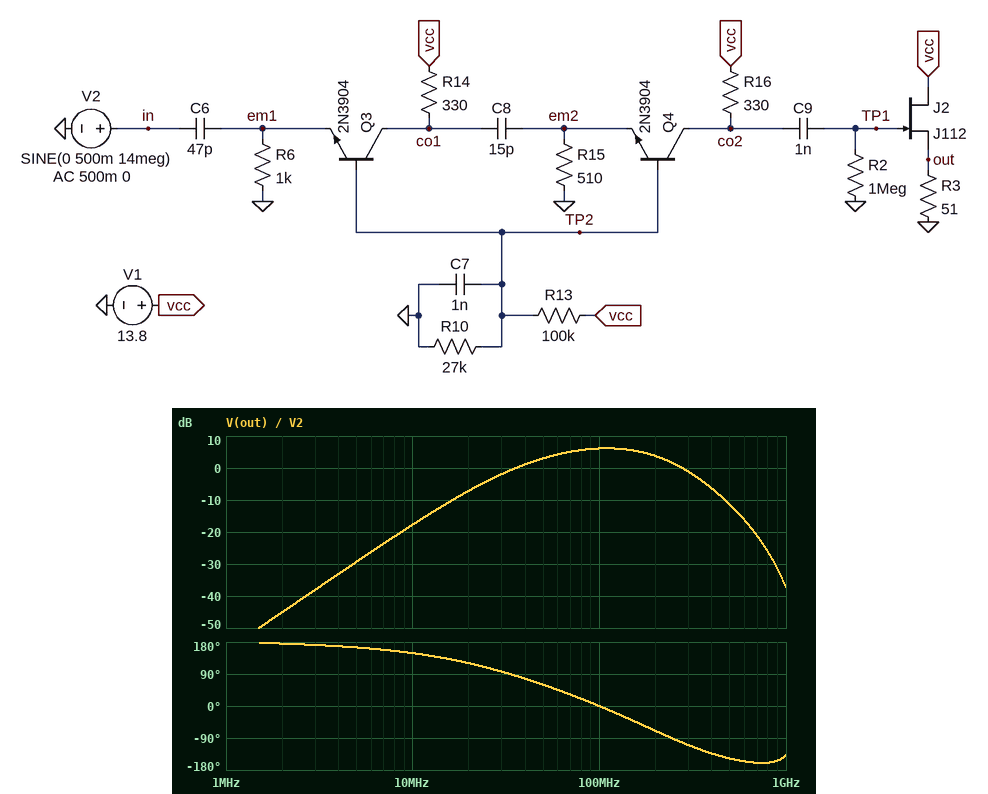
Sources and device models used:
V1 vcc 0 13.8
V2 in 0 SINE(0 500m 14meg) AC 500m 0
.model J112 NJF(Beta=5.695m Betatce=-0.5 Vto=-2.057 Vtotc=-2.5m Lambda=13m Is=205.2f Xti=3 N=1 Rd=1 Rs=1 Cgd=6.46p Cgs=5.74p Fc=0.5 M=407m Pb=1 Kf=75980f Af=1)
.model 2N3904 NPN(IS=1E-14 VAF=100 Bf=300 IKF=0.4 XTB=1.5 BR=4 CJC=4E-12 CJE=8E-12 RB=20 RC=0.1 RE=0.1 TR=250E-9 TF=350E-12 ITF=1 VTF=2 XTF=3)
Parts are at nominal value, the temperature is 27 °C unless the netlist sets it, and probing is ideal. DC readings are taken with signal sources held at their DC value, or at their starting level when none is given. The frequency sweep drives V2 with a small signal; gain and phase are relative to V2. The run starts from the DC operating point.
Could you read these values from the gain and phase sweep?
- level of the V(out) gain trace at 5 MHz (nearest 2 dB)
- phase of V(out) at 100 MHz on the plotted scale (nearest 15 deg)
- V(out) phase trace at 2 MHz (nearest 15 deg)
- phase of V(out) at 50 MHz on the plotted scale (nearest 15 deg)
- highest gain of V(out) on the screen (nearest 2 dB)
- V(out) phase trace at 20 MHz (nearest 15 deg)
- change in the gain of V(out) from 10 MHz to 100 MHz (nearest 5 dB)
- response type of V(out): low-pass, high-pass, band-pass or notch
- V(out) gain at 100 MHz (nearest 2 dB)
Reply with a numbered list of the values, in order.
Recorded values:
1. -30 dB
2. 0 deg
3. 180 deg
4. 60 deg
5. 6 dB
6. 120 deg
7. 25 dB
8. band-pass
9. 6 dB
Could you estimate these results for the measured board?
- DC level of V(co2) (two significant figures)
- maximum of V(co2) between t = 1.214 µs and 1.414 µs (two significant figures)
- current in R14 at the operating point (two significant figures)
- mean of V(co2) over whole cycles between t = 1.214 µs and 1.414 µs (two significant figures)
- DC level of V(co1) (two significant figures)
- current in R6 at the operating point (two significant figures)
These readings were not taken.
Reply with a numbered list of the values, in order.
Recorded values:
1. 13 V
2. 13 V
3. 1.9 mA
4. 13 V
5. 13 V
6. 1.9 mA
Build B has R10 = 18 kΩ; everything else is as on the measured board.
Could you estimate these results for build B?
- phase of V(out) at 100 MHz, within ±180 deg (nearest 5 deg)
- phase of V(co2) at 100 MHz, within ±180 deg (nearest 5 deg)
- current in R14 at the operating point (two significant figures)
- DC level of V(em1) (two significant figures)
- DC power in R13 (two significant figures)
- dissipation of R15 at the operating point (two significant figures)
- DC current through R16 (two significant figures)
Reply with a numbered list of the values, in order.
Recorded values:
1. -10 deg
2. -15 deg
3. 1.3 mA
4. 1.3 V
5. 1.4 mW
6. 3.1 mW
7. 2.5 mA
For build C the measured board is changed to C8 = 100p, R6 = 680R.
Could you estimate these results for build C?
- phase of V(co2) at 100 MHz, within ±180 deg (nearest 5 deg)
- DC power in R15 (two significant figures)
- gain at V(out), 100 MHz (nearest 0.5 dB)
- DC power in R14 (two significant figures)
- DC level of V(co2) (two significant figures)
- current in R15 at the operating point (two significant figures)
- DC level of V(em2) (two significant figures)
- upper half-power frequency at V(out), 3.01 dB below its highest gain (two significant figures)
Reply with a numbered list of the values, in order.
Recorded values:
1. -10 deg
2. 6.6 mW
3. 8.0 dB
4. 2.4 mW
5. 13 V
6. 3.6 mA
7. 1.8 V
8. 240 MHz
